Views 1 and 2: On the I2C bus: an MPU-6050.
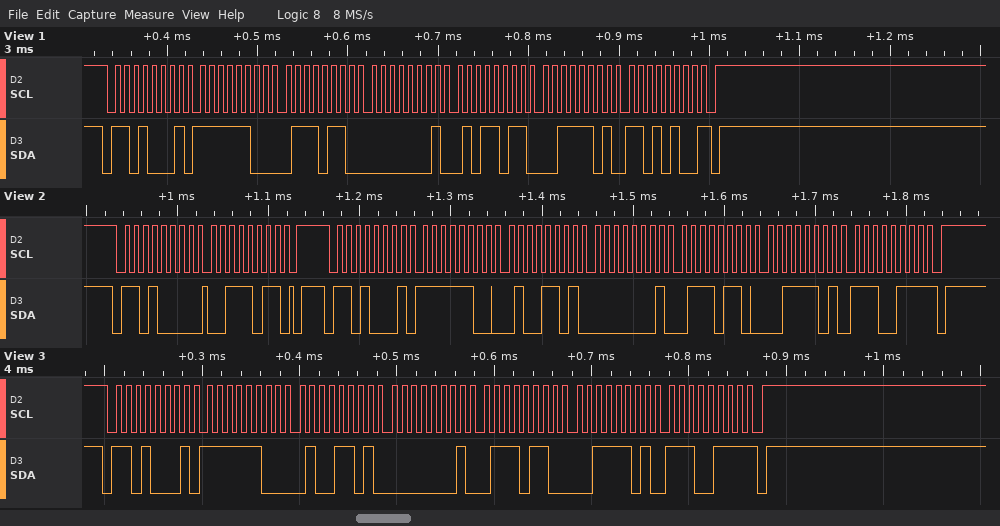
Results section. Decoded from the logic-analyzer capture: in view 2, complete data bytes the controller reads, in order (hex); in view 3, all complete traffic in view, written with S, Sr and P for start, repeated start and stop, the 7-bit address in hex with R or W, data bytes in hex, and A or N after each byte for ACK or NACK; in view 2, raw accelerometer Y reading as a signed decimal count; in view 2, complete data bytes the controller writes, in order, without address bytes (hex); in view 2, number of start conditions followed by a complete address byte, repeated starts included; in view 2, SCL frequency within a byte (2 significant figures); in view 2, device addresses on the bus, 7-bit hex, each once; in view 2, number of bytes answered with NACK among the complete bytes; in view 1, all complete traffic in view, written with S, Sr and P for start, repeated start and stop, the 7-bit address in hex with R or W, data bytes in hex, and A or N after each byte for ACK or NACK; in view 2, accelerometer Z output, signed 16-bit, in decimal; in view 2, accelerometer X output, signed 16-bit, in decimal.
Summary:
FC 4D 01 76 3D E7
S 68R A FC A 4D A 01 A 76 A 3D A E7 N P
374
3B
2
100 kHz
0x68
1
S 68R A FC A 76 A 01 A 5B A 3D A D4 N P
15847
-947
